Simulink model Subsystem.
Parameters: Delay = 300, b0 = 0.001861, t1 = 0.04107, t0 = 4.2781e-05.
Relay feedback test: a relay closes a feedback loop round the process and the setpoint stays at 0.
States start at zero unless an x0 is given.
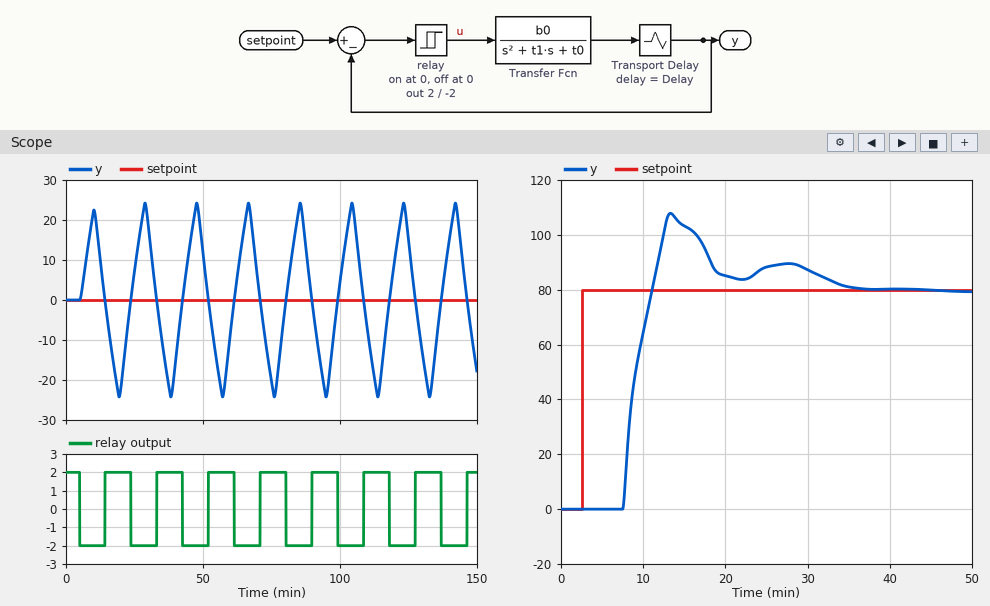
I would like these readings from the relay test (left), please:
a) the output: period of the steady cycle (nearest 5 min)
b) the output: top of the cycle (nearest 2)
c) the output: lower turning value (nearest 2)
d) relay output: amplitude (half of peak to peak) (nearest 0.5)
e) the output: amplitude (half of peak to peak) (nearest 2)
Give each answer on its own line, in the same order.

20 min
24
-24
2.0
24
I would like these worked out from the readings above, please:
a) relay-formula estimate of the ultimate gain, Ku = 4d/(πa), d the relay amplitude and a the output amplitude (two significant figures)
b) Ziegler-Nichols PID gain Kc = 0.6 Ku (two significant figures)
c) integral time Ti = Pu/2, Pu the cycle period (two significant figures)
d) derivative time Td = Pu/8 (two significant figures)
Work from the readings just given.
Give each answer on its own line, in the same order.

0.11
0.066
10 min
2.5 min
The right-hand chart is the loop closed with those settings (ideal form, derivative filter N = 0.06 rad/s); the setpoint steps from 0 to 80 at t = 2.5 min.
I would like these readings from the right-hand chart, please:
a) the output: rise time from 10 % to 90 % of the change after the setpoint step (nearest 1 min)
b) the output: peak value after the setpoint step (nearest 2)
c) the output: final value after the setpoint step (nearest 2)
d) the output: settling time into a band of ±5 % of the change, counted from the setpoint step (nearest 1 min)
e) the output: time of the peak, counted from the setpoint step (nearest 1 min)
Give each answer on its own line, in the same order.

3 min
108
80
30 min
11 min
